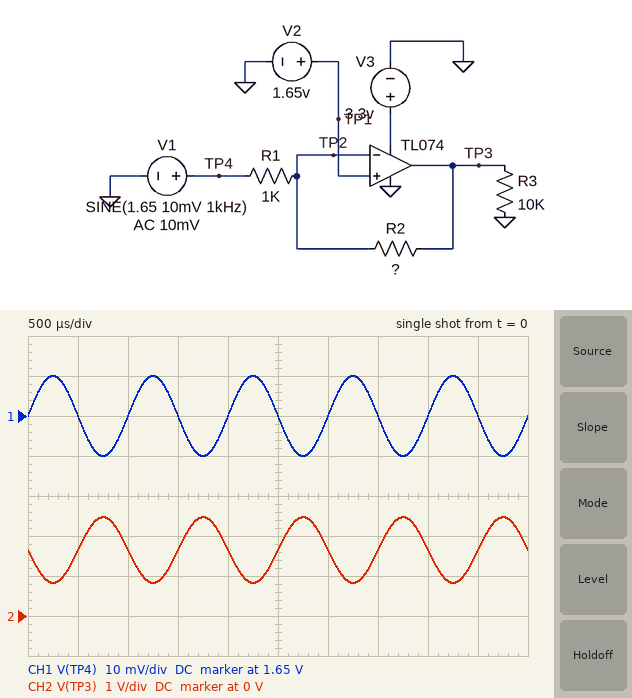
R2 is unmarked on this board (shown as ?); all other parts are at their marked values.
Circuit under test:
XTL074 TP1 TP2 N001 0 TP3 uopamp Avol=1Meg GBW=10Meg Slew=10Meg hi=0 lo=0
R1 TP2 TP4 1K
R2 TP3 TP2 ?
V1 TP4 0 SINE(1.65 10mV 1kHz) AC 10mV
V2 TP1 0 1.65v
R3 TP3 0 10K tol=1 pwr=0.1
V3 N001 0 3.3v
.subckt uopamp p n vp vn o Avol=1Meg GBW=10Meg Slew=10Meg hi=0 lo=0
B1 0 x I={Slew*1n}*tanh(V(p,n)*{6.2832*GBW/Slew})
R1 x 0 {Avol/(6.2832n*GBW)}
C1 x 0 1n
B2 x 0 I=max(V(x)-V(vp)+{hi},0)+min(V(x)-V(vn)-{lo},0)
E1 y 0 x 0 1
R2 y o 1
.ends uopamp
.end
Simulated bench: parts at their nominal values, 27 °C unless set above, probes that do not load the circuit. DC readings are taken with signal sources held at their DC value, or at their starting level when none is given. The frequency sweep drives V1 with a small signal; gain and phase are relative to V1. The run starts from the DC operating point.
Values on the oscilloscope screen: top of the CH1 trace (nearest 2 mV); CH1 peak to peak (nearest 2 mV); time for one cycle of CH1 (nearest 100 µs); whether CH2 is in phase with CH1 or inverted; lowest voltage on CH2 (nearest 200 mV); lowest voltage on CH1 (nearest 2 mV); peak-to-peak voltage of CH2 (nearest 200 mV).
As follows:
1.660 V
20 mV
1.0 ms
inverted
800 mV
1.640 V
1.6 V
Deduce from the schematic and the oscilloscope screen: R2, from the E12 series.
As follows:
82 kΩ
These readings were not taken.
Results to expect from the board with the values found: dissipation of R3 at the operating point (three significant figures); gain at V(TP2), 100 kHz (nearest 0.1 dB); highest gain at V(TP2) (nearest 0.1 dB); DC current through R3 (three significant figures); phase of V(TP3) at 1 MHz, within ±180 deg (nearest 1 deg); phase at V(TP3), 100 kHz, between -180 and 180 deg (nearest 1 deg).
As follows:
272 µW
-4.0 dB
-0.1 dB
165 µA
97 deg
140 deg
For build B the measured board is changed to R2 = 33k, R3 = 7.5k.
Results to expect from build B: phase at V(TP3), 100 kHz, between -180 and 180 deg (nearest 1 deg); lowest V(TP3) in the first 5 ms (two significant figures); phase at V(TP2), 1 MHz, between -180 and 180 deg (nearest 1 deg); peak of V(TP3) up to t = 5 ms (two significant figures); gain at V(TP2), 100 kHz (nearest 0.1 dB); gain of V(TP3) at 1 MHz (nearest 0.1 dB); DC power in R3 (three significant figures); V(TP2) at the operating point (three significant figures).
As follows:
161 deg
1.3 V
16 deg
2.0 V
-10.1 dB
19.4 dB
363 µW
1.65 V
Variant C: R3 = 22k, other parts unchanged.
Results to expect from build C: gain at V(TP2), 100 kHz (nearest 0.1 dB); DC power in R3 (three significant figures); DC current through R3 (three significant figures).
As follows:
-4.0 dB
124 µW
75.0 µA
